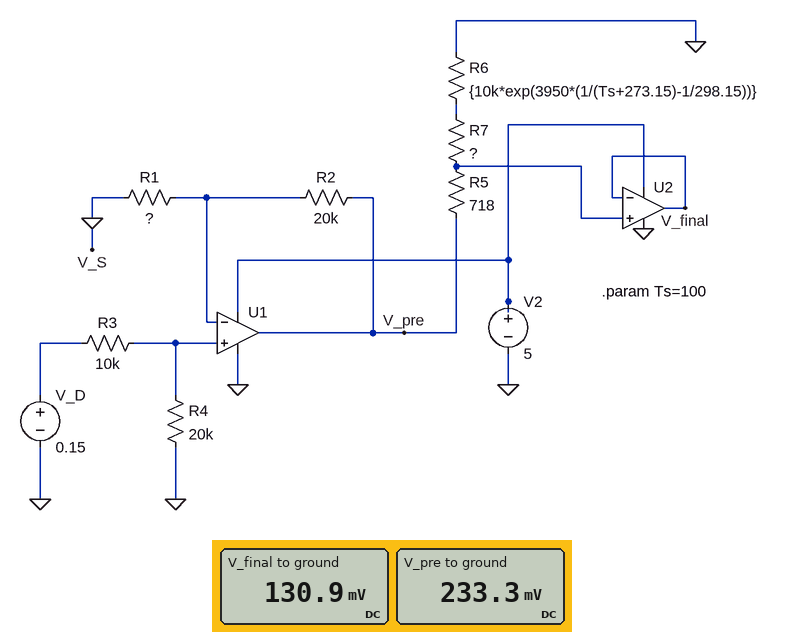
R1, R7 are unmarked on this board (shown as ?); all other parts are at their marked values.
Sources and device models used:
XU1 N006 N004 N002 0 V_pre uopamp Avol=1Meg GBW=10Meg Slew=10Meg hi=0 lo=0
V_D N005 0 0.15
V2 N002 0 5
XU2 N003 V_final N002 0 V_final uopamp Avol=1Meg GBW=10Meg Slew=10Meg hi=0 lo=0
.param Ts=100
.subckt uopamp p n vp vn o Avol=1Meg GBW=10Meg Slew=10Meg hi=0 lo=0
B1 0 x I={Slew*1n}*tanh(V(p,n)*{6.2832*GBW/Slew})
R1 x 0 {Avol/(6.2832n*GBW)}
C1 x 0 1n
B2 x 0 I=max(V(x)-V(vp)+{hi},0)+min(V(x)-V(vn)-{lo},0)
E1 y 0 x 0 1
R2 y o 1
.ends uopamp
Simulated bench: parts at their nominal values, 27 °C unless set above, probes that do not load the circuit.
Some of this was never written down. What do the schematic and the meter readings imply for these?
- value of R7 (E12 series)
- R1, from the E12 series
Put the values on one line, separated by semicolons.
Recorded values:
220 Ω; 15 kΩ
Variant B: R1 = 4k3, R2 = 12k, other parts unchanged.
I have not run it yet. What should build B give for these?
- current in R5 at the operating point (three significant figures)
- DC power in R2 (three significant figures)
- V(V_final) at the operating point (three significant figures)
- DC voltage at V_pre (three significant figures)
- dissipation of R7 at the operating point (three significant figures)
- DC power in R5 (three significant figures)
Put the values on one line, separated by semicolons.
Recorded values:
232 µA; 6.49 µW; 213 mV; 379 mV; 11.8 µW; 38.6 µW
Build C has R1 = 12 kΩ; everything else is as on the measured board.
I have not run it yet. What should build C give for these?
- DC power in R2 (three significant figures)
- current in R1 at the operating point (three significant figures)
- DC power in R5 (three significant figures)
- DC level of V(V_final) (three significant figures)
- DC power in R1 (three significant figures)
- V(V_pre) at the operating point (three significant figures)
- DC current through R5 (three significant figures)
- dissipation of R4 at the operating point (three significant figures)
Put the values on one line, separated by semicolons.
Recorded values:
1.39 µW; 8.33 µA; 19.1 µW; 150 mV; 833 nW; 267 mV; 163 µA; 500 nW
